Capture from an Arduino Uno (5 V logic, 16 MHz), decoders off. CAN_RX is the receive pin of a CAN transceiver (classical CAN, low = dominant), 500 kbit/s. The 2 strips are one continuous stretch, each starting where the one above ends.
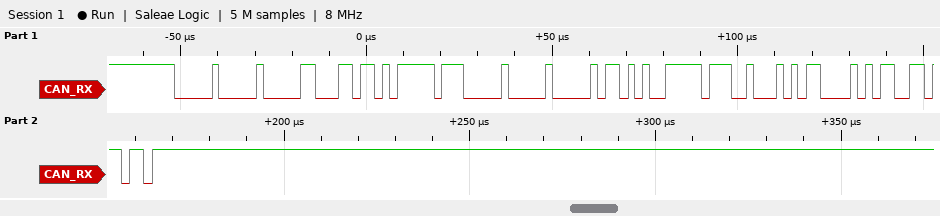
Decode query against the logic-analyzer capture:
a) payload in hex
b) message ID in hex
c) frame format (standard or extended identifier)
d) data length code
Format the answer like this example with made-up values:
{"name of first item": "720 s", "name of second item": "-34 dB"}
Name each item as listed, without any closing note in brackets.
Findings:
{"payload in hex": "DA FF 00 00 D4 FF 22 B0", "message ID in hex": "0x000", "frame format": "standard", "data length code": "8"}
